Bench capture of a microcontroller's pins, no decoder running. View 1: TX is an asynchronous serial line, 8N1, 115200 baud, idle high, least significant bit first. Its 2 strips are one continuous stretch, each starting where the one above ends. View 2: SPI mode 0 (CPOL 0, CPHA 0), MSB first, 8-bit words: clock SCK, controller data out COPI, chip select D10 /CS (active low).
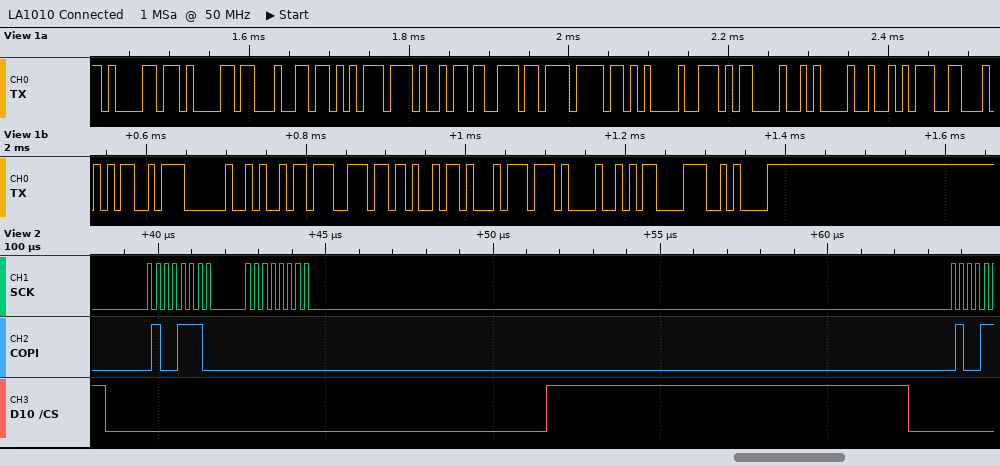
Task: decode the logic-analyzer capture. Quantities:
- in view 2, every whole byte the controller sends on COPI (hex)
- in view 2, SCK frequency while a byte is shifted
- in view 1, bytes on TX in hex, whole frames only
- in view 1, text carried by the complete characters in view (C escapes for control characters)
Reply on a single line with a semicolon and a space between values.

4E 00; 4 MHz; 0x61 0x61 0x64 0x75 0x69 0x6E 0x6F 0x21 0x0D 0x0A 0x52 0x46 0x4D 0x20 0x69 0x6E 0x69 0x74 0x21 0x0D 0x0A; "aaduino!\r\nRFM init!\r\n"
